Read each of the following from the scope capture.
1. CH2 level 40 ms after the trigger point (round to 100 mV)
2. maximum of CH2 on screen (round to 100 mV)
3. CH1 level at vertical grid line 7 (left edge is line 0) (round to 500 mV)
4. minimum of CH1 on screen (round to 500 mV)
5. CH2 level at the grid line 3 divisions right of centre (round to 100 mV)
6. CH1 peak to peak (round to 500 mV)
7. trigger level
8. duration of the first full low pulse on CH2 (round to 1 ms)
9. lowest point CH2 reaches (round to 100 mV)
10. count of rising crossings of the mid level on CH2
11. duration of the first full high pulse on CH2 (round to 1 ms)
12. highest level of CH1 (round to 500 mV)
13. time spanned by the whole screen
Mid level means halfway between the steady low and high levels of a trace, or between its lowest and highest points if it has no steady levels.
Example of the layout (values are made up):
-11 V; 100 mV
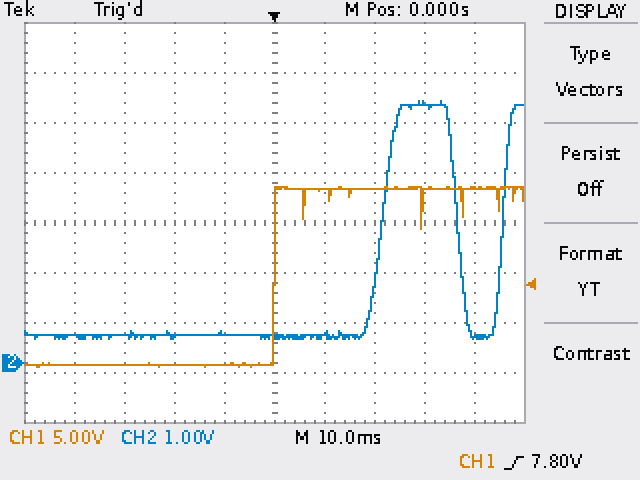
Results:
600 mV; 5.2 V; 17.5 V; -500 mV; 5.2 V; 18.0 V; 7.80 V; 9 ms; 500 mV; 2; 15 ms; 17.5 V; 100 ms
